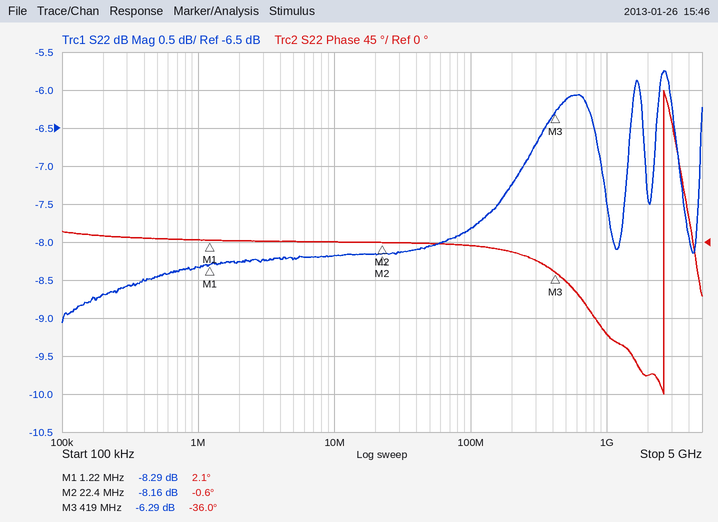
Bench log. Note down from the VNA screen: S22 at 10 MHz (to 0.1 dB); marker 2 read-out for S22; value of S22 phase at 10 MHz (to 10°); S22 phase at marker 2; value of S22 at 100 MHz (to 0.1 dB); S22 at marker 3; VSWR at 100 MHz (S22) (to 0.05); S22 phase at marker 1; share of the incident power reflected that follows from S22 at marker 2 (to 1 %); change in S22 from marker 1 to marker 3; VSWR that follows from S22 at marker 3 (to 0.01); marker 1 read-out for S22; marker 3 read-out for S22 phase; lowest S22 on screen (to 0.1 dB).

-8.2 dB
-8.16 dB
0°
-0.6°
-7.8 dB
-6.29 dB
2.35
2.1°
15 %
2.00 dB
2.88
-8.29 dB
-36.0°
-9.1 dB
